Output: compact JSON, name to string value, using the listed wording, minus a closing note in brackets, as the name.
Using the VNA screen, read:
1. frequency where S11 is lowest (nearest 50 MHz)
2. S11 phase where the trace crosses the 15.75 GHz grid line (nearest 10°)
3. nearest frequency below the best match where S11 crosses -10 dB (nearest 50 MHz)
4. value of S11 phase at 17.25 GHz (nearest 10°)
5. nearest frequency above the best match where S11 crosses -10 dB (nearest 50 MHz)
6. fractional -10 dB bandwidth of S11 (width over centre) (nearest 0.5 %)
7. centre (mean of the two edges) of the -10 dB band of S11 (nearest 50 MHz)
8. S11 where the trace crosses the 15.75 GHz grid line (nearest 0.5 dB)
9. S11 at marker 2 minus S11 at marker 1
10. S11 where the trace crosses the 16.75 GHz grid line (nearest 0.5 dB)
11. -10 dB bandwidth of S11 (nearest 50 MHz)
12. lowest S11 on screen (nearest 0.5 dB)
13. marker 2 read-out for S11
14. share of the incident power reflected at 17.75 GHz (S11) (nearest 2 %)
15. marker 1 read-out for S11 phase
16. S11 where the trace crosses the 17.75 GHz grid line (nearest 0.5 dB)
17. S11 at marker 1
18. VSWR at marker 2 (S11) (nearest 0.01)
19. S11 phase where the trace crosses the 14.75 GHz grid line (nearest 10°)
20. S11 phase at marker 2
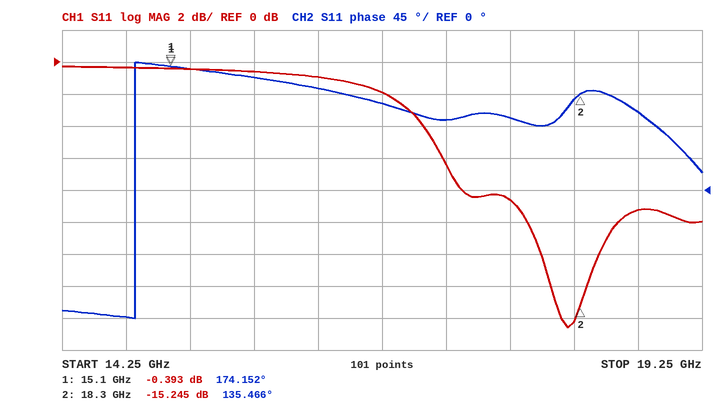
{"frequency where S11 is lowest": "18.20 GHz", "S11 phase where the trace crosses the 15.75 GHz grid line": "160°", "nearest frequency below the best match where S11 crosses -10 dB": "17.90 GHz", "value of S11 phase at 17.25 GHz": "100°", "nearest frequency above the best match where S11 crosses -10 dB": "18.60 GHz", "fractional -10 dB bandwidth of S11 (width over centre)": "4.0 %", "centre (mean of the two edges) of the -10 dB band of S11": "18.25 GHz", "S11 where the trace crosses the 15.75 GHz grid line": "-0.5 dB", "S11 at marker 2 minus S11 at marker 1": "-14.852 dB", "S11 where the trace crosses the 16.75 GHz grid line": "-2.0 dB", "-10 dB bandwidth of S11": "700 MHz", "lowest S11 on screen": "-16.5 dB", "marker 2 read-out for S11": "-15.245 dB", "share of the incident power reflected at 17.75 GHz (S11)": "14 %", "marker 1 read-out for S11 phase": "174.152°", "S11 where the trace crosses the 17.75 GHz grid line": "-8.5 dB", "S11 at marker 1": "-0.393 dB", "VSWR at marker 2 (S11)": "1.42", "S11 phase where the trace crosses the 14.75 GHz grid line": "-180°", "S11 phase at marker 2": "135.466°"}
